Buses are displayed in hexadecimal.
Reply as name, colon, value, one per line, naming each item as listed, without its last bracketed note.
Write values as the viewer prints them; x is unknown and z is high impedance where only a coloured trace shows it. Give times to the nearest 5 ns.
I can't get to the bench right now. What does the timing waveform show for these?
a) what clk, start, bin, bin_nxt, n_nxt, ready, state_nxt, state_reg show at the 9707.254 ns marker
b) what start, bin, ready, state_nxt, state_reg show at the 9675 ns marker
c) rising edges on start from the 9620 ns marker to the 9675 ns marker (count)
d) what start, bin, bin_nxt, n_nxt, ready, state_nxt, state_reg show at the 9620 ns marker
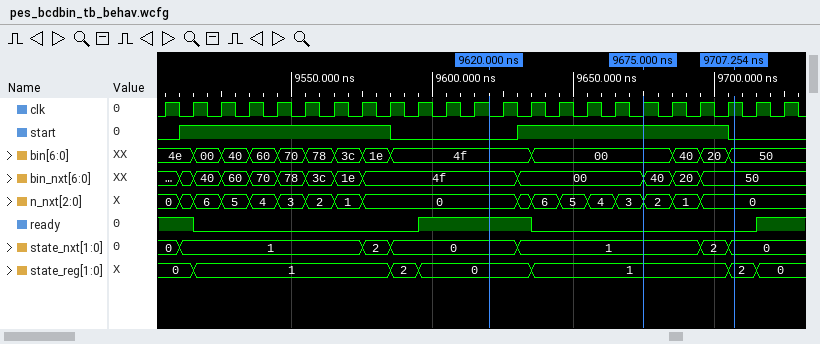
what clk, start, bin, bin_nxt, n_nxt, ready, state_nxt, state_reg show at the 9707.254 ns marker: clk=1, start=0, bin=50, bin_nxt=50, n_nxt=0, ready=0, state_nxt=0, state_reg=2
what start, bin, ready, state_nxt, state_reg show at the 9675 ns marker: start=1, bin=00, ready=0, state_nxt=1, state_reg=1
rising edges on start from the 9620 ns marker to the 9675 ns marker: 1
what start, bin, bin_nxt, n_nxt, ready, state_nxt, state_reg show at the 9620 ns marker: start=0, bin=4f, bin_nxt=4f, n_nxt=0, ready=1, state_nxt=0, state_reg=0
